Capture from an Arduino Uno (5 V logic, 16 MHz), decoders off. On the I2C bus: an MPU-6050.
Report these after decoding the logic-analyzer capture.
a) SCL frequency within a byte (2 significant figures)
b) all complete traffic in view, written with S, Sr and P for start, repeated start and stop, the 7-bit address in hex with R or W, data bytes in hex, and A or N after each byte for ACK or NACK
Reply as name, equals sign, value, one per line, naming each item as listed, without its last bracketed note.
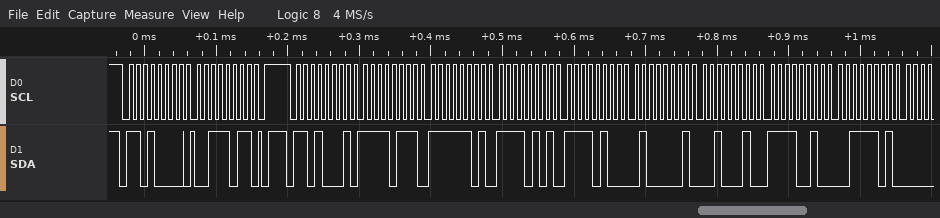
SCL frequency within a byte = 100 kHz
all complete traffic in view, written with S, Sr and P for start, repeated start and stop, the 7-bit address in hex with R or W, data bytes in hex, and A or N after each byte for ACK or NACK = S 68W A 3B A P S 68R A F7 A FD A F5 A F4 A 41 A 22 A F2 A 3D A
